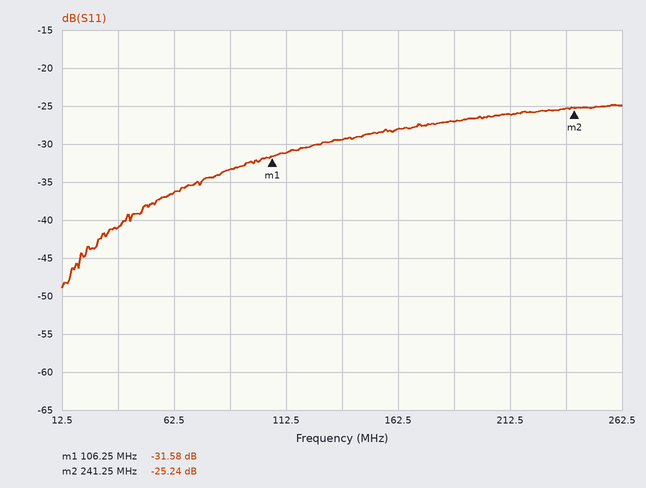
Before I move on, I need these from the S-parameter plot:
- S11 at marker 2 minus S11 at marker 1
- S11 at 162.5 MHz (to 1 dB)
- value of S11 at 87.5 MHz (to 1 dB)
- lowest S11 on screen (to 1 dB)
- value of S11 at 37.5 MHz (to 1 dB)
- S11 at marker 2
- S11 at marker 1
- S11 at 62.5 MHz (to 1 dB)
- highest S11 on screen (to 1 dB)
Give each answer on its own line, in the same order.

6.34 dB
-28 dB
-33 dB
-49 dB
-41 dB
-25.24 dB
-31.58 dB
-36 dB
-25 dB
